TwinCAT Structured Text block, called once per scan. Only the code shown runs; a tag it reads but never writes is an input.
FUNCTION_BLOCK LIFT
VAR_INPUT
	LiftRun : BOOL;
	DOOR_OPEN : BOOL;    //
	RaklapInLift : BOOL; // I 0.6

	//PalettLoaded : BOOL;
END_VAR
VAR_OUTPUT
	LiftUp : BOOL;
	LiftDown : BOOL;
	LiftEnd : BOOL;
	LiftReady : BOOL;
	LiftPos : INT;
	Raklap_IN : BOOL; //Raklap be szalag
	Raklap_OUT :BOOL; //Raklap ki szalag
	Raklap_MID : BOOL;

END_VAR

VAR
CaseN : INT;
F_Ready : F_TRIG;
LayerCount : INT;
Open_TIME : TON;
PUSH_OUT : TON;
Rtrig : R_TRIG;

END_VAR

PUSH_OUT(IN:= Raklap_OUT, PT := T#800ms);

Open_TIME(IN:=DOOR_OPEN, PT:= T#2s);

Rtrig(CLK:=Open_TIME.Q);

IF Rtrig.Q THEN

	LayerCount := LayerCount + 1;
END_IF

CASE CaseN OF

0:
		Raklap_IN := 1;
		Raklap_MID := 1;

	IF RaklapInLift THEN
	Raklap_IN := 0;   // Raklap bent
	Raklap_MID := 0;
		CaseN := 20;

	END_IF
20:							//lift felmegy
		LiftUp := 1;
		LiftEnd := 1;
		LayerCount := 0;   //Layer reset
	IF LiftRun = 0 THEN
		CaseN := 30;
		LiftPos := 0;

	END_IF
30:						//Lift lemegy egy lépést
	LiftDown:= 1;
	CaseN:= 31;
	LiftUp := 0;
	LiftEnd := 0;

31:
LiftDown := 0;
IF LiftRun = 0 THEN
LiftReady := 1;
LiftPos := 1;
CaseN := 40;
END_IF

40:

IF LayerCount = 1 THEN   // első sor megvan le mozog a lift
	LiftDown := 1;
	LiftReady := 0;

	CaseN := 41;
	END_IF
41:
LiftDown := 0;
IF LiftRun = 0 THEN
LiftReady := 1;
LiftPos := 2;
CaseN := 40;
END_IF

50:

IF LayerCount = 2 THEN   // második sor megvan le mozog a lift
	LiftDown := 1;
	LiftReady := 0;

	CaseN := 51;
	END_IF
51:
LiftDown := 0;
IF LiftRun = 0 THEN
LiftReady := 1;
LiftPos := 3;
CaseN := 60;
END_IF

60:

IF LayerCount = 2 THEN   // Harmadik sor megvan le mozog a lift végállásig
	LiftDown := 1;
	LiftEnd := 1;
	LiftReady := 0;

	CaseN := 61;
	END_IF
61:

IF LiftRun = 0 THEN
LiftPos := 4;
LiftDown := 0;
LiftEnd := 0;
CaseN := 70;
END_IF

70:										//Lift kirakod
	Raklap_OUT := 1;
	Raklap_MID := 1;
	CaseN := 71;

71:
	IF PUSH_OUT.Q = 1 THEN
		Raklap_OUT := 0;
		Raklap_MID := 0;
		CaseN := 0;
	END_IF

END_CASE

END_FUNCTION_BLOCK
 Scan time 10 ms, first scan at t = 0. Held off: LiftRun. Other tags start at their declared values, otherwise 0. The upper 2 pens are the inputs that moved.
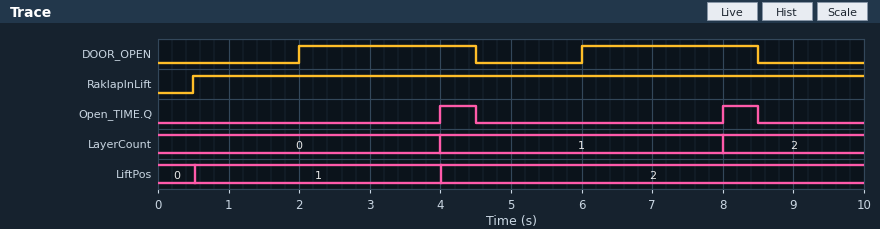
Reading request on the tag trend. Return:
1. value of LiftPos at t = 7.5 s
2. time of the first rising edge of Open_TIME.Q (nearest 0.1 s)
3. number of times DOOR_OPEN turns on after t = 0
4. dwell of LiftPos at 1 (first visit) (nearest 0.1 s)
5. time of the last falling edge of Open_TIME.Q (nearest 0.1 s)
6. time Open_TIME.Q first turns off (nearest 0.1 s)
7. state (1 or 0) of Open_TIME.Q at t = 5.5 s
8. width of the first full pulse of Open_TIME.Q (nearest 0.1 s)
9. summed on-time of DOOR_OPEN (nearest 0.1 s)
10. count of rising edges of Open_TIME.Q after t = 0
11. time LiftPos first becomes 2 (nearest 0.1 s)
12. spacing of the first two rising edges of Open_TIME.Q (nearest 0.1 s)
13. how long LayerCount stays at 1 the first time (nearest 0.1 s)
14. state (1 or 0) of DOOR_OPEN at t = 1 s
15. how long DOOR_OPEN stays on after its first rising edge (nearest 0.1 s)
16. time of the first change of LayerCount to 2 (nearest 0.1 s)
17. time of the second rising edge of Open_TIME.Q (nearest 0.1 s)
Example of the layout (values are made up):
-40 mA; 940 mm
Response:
2; 4.0 s; 2; 3.5 s; 8.5 s; 4.5 s; 0; 0.5 s; 5.0 s; 2; 4.0 s; 4.0 s; 4.0 s; 0; 2.5 s; 8.0 s; 8.0 s
